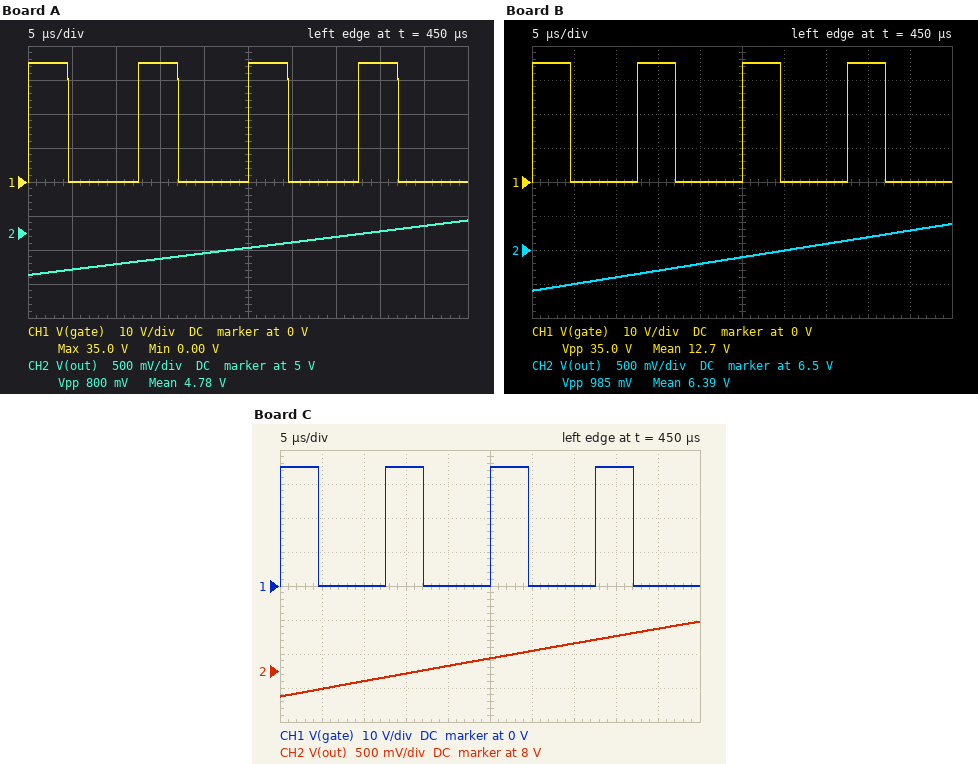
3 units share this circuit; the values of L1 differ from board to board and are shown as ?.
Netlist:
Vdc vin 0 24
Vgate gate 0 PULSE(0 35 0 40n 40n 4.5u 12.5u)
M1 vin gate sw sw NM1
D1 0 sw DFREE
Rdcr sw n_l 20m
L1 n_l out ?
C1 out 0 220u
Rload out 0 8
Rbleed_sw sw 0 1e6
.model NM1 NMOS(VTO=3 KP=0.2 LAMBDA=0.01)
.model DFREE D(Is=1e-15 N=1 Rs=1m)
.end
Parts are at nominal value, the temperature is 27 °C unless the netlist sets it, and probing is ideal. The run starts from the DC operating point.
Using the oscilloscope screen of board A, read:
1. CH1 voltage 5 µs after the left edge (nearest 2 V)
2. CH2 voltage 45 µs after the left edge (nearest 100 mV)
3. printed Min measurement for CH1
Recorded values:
0 V
5.1 V
0.00 V
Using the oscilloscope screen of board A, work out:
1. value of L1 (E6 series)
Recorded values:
680 µH
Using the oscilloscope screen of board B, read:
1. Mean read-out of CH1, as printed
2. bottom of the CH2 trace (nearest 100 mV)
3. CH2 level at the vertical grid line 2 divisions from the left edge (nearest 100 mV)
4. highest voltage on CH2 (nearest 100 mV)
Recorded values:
12.7 V
5.9 V
6.1 V
6.9 V
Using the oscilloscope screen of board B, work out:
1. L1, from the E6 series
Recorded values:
470 µH
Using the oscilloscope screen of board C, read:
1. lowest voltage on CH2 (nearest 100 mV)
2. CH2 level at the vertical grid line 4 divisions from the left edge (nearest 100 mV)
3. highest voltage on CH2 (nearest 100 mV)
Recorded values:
7.6 V
8.1 V
8.7 V
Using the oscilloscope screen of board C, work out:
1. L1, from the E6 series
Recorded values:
330 µH
